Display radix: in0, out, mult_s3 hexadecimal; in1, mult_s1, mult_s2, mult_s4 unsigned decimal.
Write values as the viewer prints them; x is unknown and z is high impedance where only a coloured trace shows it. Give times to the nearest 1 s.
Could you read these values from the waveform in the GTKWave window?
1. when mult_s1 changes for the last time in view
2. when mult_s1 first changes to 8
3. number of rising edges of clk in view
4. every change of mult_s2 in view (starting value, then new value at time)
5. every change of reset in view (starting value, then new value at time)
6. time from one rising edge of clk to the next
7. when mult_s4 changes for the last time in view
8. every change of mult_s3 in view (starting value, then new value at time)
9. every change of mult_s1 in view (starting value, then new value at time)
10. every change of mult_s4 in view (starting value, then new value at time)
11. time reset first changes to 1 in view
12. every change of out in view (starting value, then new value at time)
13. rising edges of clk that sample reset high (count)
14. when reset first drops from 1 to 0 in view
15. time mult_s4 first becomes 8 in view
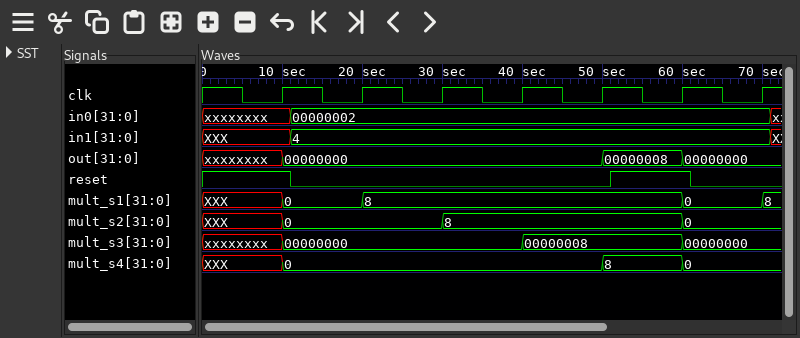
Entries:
70 s
20 s
7
XXX, 0 at 10 s, 8 at 30 s, 0 at 60 s
1, 0 at 11 s, 1 at 51 s, 0 at 61 s
10 s
60 s
xxxxxxxx, 00000000 at 10 s, 00000008 at 40 s, 00000000 at 60 s
XXX, 0 at 10 s, 8 at 20 s, 0 at 60 s, 8 at 70 s
XXX, 0 at 10 s, 8 at 50 s, 0 at 60 s
51 s
xxxxxxxx, 00000000 at 10 s, 00000008 at 50 s, 00000000 at 60 s
2
11 s
50 s
